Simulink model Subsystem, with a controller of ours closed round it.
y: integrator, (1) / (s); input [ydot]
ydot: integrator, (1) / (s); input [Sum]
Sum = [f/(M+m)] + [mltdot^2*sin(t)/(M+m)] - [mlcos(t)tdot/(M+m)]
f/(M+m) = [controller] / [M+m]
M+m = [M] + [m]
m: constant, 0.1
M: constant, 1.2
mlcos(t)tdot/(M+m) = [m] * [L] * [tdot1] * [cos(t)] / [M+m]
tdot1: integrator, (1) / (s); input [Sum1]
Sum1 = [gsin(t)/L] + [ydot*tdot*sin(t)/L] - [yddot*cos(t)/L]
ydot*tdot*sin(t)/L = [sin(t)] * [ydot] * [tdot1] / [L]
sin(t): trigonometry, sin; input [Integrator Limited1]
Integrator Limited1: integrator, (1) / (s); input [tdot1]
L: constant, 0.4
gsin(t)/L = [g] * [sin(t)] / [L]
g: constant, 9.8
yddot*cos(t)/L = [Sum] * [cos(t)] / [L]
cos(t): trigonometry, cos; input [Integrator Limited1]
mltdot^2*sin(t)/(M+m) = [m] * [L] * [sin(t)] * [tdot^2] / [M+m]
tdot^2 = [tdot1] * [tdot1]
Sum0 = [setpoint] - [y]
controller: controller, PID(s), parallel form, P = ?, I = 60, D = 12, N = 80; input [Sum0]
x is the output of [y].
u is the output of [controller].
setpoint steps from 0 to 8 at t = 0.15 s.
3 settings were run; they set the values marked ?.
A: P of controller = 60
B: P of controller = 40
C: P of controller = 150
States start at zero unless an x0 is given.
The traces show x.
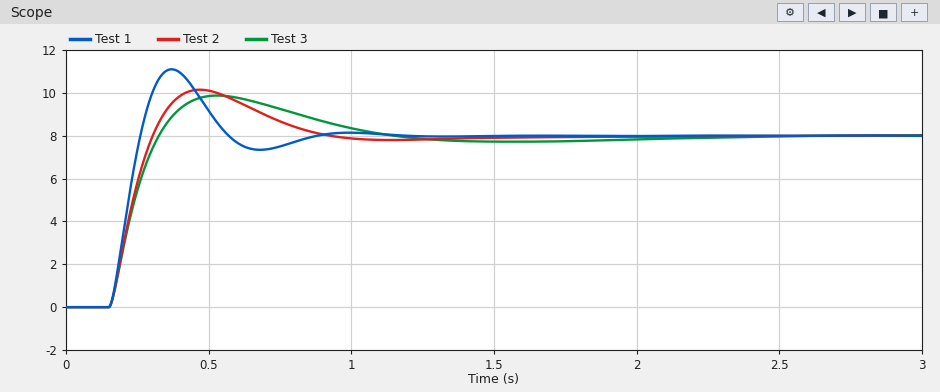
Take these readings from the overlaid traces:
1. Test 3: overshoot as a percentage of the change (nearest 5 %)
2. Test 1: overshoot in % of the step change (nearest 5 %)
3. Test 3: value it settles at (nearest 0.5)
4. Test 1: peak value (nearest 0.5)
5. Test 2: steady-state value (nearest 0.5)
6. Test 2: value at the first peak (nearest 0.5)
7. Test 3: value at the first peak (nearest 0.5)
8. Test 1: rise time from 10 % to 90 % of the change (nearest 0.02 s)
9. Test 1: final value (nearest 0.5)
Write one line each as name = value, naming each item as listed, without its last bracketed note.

Test 3: overshoot as a percentage of the change = 25 %
Test 1: overshoot in % of the step change = 40 %
Test 3: value it settles at = 8.0
Test 1: peak value = 11.0
Test 2: steady-state value = 8.0
Test 2: value at the first peak = 10.0
Test 3: value at the first peak = 10.0
Test 1: rise time from 10 % to 90 % of the change = 0.08 s
Test 1: final value = 8.0
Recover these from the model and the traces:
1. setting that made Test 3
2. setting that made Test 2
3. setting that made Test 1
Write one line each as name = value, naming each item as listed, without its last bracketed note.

setting that made Test 3 = B
setting that made Test 2 = A
setting that made Test 1 = C
